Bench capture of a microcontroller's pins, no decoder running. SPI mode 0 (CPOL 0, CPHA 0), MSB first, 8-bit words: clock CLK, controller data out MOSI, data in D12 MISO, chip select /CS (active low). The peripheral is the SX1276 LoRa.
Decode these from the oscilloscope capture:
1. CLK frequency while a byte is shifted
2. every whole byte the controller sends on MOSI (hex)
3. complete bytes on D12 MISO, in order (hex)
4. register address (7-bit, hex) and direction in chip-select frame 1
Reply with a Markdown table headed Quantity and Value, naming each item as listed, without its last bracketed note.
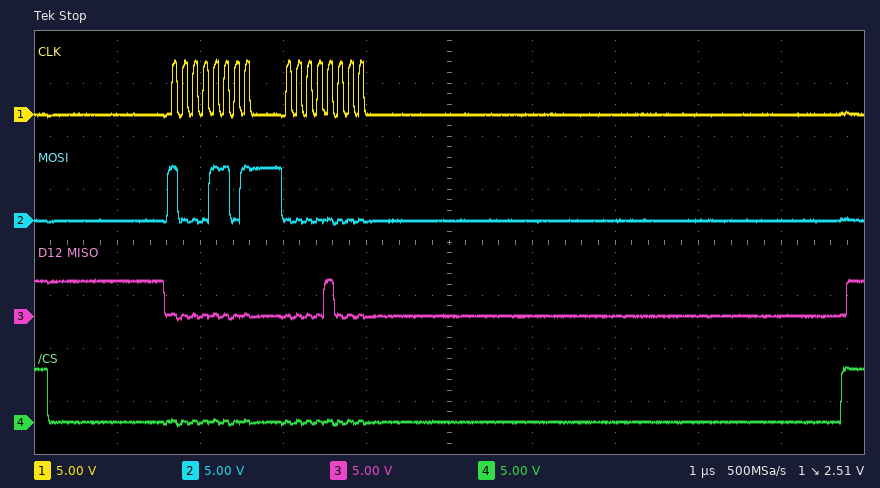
| Quantity | Value |
|---|---|
| CLK frequency while a byte is shifted | 8 MHz |
| every whole byte the controller sends on MOSI | 8D 00 |
| complete bytes on D12 MISO, in order | 00 08 |
| register address (7-bit, hex) and direction in chip-select frame 1 | 0x0D write |
